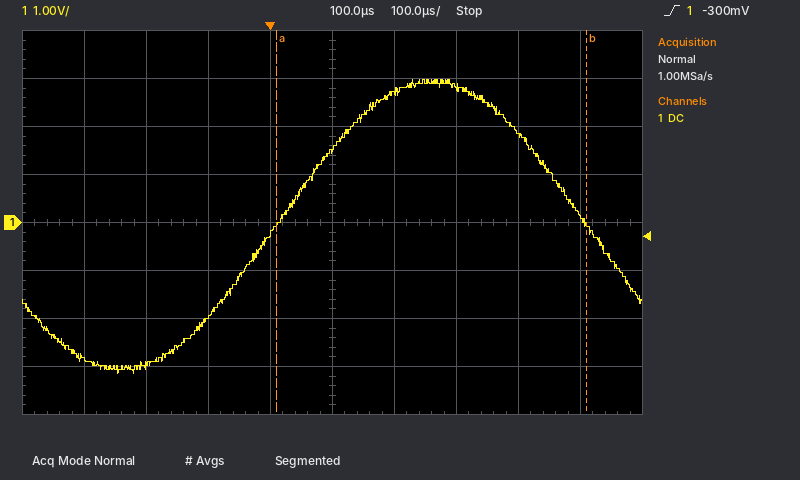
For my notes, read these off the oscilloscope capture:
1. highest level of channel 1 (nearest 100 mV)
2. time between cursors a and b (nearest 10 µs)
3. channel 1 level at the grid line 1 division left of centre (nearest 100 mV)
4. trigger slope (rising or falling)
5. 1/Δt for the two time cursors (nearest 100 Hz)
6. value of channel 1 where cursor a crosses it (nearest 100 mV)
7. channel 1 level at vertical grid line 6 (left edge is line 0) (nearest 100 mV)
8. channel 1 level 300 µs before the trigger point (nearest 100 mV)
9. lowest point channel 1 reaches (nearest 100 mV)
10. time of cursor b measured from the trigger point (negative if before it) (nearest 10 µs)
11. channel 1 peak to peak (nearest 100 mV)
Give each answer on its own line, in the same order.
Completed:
3.0 V
500 µs
-200 mV
rising
2.0 kHz
-100 mV
2.7 V
-2.8 V
-3.1 V
+510 µs
6.1 V
